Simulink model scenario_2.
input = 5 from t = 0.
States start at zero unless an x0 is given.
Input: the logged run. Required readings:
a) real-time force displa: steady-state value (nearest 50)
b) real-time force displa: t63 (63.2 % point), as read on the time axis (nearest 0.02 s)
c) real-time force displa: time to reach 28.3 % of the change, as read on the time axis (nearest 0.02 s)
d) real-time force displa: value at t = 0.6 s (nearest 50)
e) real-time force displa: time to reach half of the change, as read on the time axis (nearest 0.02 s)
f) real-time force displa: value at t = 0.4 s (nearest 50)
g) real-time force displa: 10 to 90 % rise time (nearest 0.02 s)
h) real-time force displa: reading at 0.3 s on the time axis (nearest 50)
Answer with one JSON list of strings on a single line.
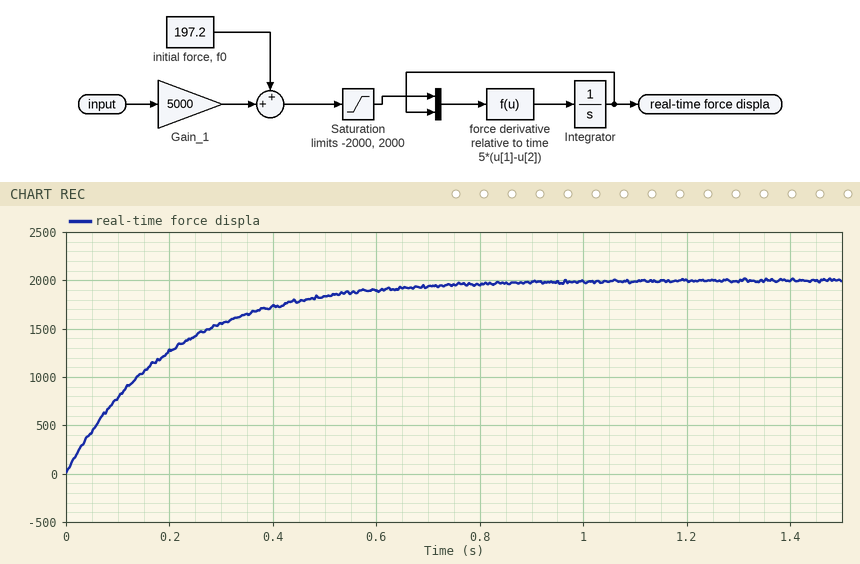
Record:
["2000", "0.20 s", "0.06 s", "1900", "0.14 s", "1750", "0.44 s", "1550"]
